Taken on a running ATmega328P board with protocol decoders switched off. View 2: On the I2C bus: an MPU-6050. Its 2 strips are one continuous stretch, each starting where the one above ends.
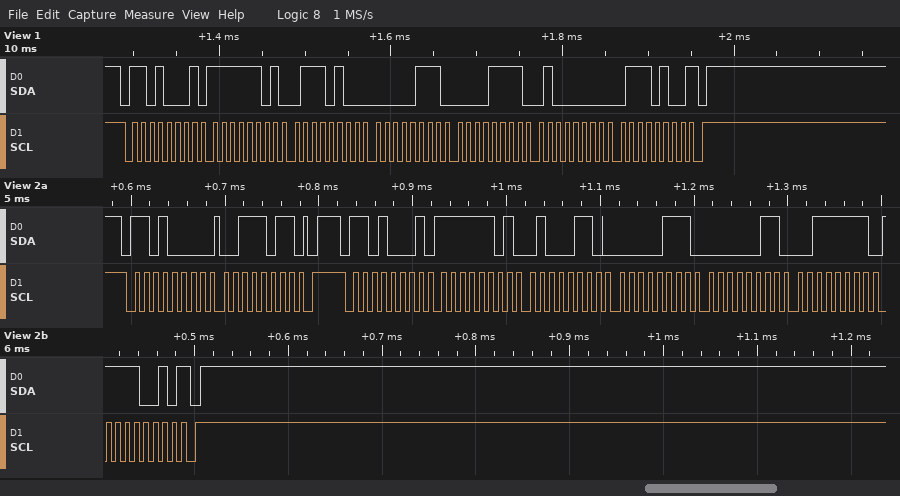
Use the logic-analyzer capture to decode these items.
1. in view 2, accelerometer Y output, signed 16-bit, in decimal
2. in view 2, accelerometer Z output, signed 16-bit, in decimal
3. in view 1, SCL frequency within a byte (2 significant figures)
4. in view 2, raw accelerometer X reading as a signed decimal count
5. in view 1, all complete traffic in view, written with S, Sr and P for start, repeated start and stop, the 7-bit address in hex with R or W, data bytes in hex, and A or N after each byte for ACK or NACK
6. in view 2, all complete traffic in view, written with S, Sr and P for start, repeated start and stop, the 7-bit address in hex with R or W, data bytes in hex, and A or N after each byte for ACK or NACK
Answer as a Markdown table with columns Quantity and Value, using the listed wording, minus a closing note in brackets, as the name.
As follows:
| Quantity | Value |
|---|---|
| in view 2, accelerometer Y output, signed 16-bit, in decimal | 1795 |
| in view 2, accelerometer Z output, signed 16-bit, in decimal | 16370 |
| in view 1, SCL frequency within a byte | 100 kHz |
| in view 2, raw accelerometer X reading as a signed decimal count | -698 |
| in view 1, all complete traffic in view, written with S, Sr and P for start, repeated start and stop, the 7-bit address in hex with R or W, data bytes in hex, and A or N after each byte for ACK or NACK | S 68R A FD A 74 A 07 A 0F A 40 A 74 N P |
| in view 2, all complete traffic in view, written with S, Sr and P for start, repeated start and stop, the 7-bit address in hex with R or W, data bytes in hex, and A or N after each byte for ACK or NACK | S 68W A 3B A P S 68R A FD A 46 A 07 A 03 A 3F A F2 N P |
